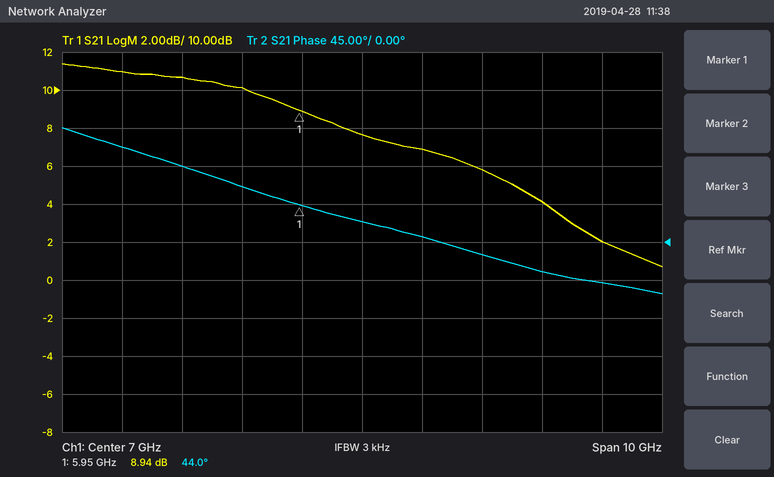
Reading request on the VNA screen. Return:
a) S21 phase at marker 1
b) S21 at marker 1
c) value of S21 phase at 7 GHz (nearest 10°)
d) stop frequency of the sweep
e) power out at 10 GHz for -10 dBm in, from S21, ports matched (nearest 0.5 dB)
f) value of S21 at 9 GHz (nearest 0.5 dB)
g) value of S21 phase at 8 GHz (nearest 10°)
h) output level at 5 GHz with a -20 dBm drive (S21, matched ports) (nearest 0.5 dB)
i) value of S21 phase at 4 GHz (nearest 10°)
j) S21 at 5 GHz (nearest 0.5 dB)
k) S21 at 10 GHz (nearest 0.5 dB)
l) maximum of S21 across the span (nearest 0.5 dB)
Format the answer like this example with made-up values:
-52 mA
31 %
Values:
44.0°
8.94 dB
20°
12 GHz
-6.0 dBm
6.0 dB
10°
-10.0 dBm
90°
10.0 dB
4.0 dB
11.5 dB
